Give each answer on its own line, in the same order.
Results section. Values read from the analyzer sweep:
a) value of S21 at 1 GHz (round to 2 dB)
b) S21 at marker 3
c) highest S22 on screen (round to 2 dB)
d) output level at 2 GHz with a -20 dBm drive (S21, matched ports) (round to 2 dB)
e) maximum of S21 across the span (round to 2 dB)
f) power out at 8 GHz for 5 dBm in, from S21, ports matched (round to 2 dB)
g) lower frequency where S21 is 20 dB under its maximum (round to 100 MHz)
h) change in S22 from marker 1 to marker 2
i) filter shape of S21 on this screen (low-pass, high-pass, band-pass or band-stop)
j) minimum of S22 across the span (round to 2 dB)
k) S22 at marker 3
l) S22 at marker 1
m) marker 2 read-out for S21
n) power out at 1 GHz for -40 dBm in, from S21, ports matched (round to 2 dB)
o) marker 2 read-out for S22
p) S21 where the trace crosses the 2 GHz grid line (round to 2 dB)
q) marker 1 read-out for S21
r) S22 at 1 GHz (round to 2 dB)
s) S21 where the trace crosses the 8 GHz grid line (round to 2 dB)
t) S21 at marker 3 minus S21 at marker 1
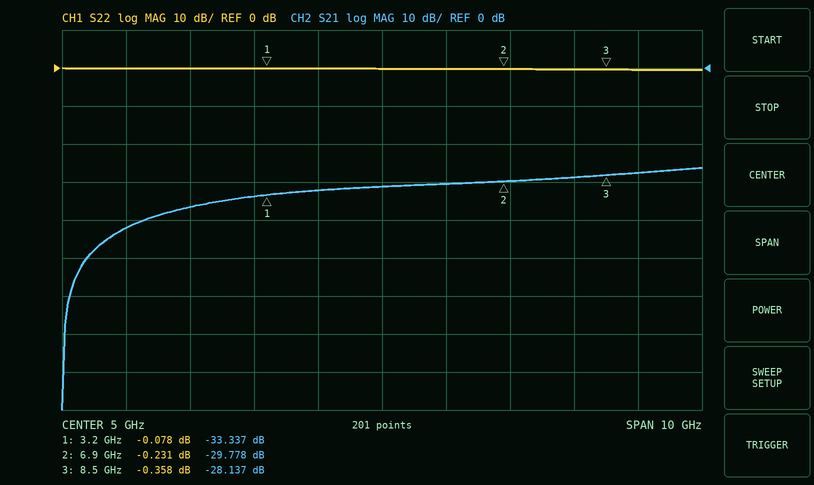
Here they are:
-42 dB
-28.137 dB
0 dB
-56 dBm
-26 dB
-24 dBm
600 MHz
-0.153 dB
high-pass
0 dB
-0.358 dB
-0.078 dB
-29.778 dB
-82 dBm
-0.231 dB
-36 dB
-33.337 dB
0 dB
-28 dB
5.200 dB
